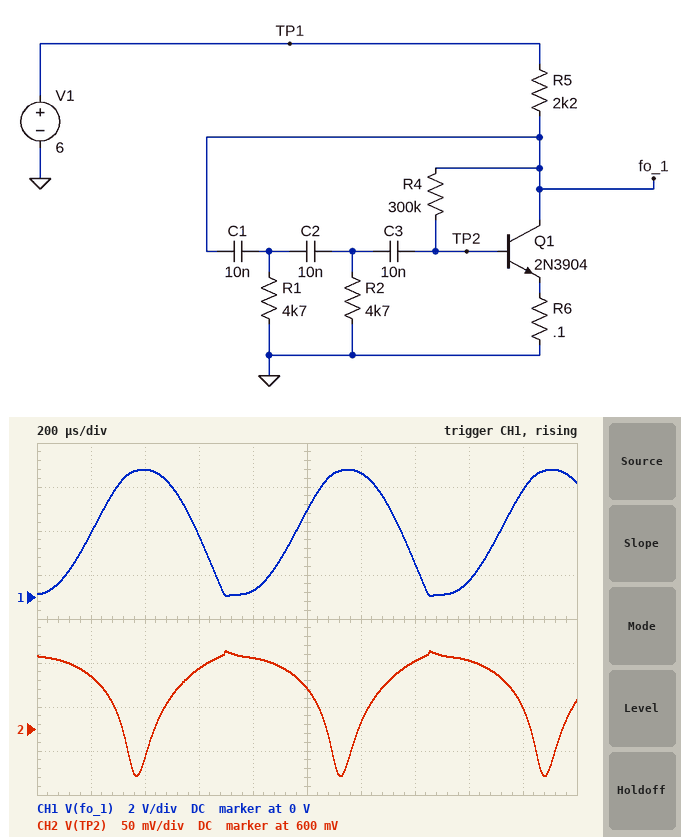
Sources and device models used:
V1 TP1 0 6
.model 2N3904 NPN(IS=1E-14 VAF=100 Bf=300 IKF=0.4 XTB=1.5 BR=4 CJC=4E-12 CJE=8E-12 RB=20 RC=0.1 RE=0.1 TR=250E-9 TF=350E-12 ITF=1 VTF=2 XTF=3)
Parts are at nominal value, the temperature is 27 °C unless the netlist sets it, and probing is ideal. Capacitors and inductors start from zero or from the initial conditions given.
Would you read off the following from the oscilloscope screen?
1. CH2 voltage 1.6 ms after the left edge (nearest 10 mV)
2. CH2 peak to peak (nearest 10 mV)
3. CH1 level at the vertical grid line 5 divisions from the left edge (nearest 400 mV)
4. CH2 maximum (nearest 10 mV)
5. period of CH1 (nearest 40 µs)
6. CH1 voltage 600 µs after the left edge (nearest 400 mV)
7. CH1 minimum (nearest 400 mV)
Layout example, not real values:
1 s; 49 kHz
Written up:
680 mV; 140 mV; 4.0 V; 690 mV; 760 µs; 2.8 V; 0 V
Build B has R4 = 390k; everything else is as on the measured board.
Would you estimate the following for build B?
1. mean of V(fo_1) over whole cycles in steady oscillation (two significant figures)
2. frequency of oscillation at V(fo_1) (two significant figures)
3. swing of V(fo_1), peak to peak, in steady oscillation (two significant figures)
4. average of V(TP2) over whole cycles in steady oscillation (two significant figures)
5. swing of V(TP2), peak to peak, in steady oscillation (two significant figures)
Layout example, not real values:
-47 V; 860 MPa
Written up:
3.2 V; 1.2 kHz; 5.8 V; 630 mV; 240 mV
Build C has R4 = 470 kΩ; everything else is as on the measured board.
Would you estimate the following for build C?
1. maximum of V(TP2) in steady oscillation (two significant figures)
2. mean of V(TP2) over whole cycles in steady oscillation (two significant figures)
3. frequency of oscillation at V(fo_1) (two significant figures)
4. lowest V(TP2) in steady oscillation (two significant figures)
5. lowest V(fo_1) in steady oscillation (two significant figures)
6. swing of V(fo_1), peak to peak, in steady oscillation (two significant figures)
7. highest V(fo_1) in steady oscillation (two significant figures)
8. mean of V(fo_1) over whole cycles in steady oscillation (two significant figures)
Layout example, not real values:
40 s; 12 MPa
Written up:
690 mV; 620 mV; 1.1 kHz; 400 mV; 74 mV; 5.8 V; 5.9 V; 3.3 V
